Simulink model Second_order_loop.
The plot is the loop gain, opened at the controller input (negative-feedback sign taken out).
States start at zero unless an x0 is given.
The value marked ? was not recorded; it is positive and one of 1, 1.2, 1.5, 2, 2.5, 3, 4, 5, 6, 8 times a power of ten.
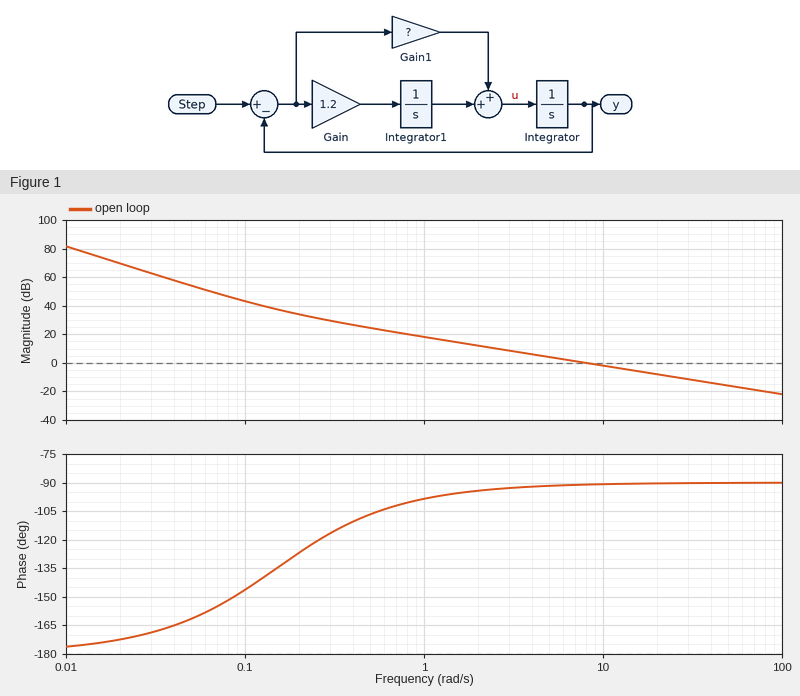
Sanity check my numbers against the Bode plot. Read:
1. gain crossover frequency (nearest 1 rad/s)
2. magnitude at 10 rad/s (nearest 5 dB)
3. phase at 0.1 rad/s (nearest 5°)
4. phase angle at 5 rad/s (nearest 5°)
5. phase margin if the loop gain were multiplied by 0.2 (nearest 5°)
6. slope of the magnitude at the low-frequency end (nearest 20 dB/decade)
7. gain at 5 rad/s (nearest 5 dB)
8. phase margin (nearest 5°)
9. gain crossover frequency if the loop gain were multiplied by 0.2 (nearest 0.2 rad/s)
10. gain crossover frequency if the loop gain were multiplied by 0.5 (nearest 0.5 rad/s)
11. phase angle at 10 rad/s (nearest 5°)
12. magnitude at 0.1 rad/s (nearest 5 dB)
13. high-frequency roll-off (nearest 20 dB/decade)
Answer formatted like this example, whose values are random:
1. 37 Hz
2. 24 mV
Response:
1. 8 rad/s
2. 0 dB
3. -145°
4. -90°
5. 85°
6. -40 dB/decade
7. 5 dB
8. 90°
9. 1.6 rad/s
10. 4.0 rad/s
11. -90°
12. 45 dB
13. -20 dB/decade
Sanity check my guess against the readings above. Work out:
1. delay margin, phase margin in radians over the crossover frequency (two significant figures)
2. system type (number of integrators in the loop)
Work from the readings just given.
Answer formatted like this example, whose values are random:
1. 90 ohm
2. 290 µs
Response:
1. 0.20 s
2. 2
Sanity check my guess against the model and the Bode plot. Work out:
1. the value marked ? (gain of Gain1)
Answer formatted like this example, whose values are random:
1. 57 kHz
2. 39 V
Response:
1. 8
